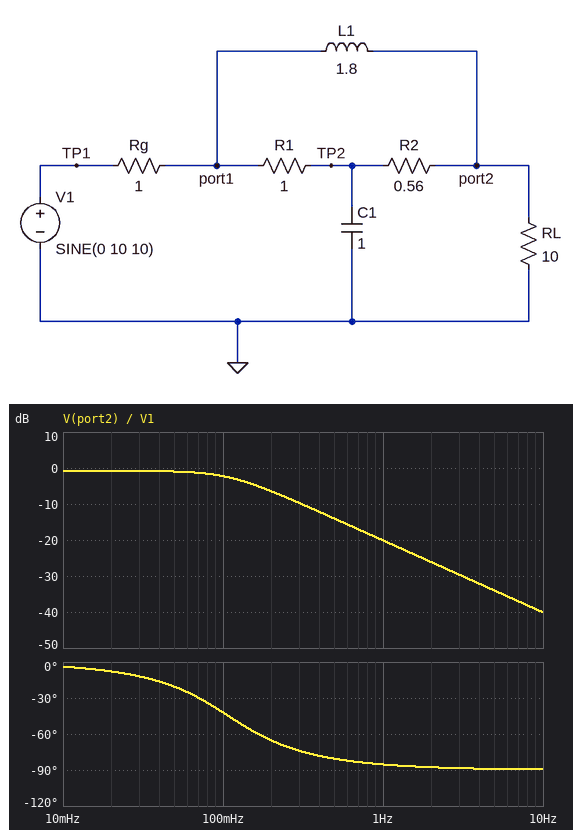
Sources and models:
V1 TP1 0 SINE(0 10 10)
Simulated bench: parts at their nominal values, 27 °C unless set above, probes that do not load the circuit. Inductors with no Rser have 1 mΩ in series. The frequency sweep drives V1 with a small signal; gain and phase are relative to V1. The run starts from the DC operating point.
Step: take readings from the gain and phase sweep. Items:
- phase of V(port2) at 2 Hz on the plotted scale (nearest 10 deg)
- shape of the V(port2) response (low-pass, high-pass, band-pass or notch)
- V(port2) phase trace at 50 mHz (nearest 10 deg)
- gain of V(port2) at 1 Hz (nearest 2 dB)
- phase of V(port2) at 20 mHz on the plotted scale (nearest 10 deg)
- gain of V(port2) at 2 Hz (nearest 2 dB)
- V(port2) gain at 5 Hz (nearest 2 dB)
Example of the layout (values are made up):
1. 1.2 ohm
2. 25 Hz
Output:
1. -90 deg
2. low-pass
3. -20 deg
4. -20 dB
5. -10 deg
6. -26 dB
7. -34 dB
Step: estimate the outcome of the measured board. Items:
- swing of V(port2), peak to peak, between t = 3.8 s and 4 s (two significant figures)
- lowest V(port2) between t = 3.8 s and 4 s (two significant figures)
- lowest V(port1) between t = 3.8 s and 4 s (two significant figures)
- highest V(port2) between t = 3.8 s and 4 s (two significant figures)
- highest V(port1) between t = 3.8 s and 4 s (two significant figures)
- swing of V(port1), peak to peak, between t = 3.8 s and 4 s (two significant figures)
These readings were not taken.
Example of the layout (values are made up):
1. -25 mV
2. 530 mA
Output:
1. 200 mV
2. -94 mV
3. -5.0 V
4. 100 mV
5. 5.0 V
6. 10 V
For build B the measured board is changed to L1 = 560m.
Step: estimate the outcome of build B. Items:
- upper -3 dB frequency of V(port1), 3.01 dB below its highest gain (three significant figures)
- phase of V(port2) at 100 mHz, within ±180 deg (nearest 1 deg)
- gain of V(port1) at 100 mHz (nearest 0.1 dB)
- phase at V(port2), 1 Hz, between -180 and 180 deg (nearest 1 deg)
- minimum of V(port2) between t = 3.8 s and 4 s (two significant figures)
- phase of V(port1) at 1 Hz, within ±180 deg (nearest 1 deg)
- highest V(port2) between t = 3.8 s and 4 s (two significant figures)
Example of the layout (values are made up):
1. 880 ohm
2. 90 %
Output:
1. 117 mHz
2. -31 deg
3. -3.2 dB
4. -81 deg
5. -150 mV
6. 3 deg
7. 150 mV
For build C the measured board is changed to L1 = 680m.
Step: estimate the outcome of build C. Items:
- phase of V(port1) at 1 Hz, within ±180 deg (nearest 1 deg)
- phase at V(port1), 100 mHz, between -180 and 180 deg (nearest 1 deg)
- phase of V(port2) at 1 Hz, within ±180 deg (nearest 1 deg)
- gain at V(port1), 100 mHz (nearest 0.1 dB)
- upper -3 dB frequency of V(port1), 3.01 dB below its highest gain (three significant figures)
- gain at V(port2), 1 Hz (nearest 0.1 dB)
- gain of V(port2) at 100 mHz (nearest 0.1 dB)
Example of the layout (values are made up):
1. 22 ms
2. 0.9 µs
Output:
1. 2 deg
2. -25 deg
3. -82 deg
4. -3.2 dB
5. 114 mHz
6. -17.3 dB
7. -2.1 dB
